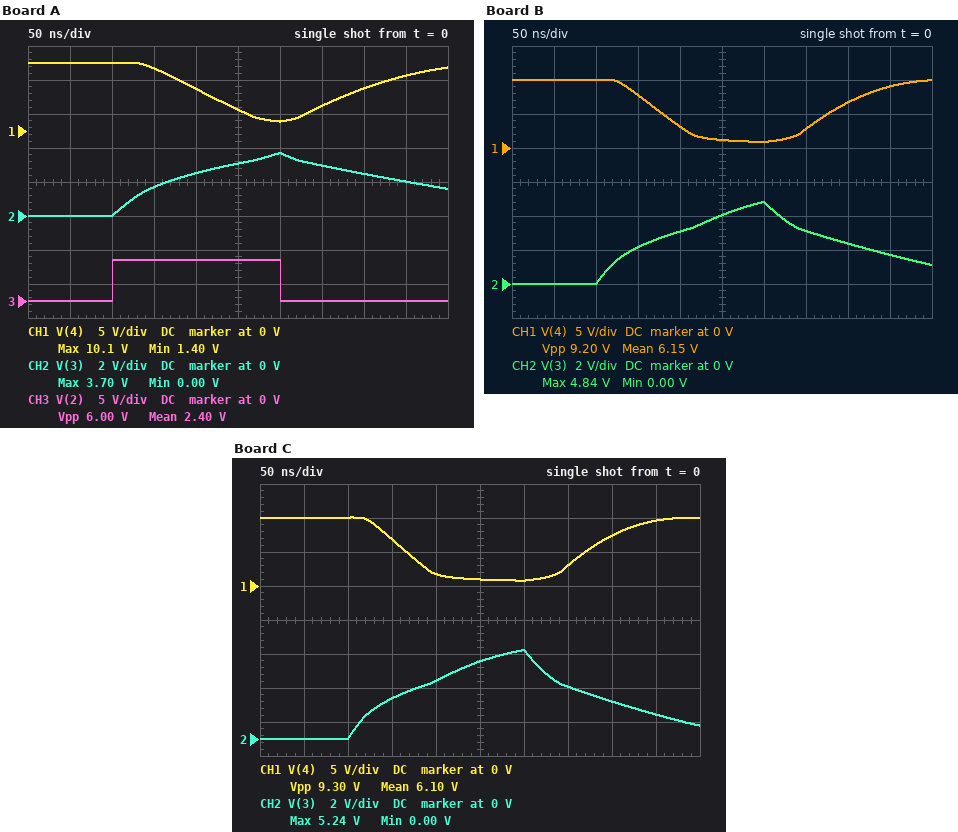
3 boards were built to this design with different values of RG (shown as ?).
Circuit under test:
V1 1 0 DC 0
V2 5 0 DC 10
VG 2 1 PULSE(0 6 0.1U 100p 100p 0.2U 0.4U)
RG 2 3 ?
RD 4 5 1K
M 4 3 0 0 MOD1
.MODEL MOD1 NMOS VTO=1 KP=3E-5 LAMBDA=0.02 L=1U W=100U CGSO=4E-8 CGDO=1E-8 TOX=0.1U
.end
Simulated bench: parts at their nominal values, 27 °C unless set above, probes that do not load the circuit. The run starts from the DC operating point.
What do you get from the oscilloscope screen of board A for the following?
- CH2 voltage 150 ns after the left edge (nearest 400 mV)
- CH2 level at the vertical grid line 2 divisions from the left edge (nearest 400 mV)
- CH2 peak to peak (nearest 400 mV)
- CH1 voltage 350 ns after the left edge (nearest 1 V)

1.6 V
0 V
3.6 V
4 V
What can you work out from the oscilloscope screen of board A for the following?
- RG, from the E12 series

27 kΩ
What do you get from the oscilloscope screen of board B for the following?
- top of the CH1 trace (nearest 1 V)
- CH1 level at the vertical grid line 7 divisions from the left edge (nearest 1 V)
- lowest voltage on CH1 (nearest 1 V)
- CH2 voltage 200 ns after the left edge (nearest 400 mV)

10 V
3 V
1 V
3.2 V
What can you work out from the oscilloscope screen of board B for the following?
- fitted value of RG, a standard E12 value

18 kΩ
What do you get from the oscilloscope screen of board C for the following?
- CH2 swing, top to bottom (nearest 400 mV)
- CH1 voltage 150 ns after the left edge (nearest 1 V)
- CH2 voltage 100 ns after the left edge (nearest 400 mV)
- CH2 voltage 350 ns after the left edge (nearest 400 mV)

5.2 V
7 V
0 V
3.2 V
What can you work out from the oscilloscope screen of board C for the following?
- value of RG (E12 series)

15 kΩ
